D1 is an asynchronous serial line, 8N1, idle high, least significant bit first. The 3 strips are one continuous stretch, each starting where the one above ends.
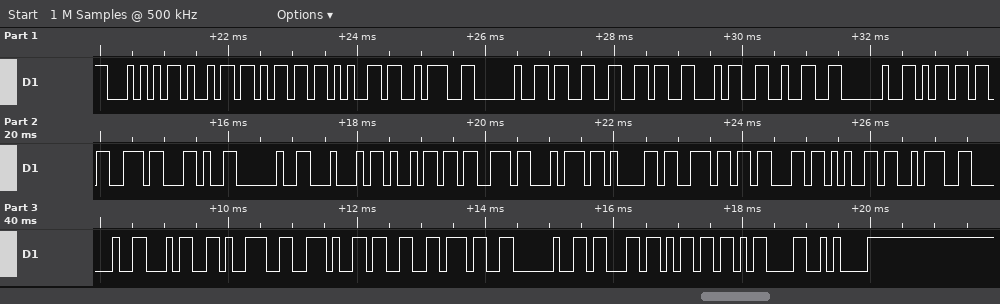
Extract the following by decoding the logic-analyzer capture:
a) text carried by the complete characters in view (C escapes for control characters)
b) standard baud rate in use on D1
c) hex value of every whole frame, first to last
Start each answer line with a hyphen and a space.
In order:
- "Time: 3642 ms, Distance: 49.37 cm\r\n"
- 9600 baud
- 54 69 6D 65 3A 20 33 36 34 32 20 6D 73 2C 20 44 69 73 74 61 6E 63 65 3A 20 34 39 2E 33 37 20 63 6D 0D 0A
